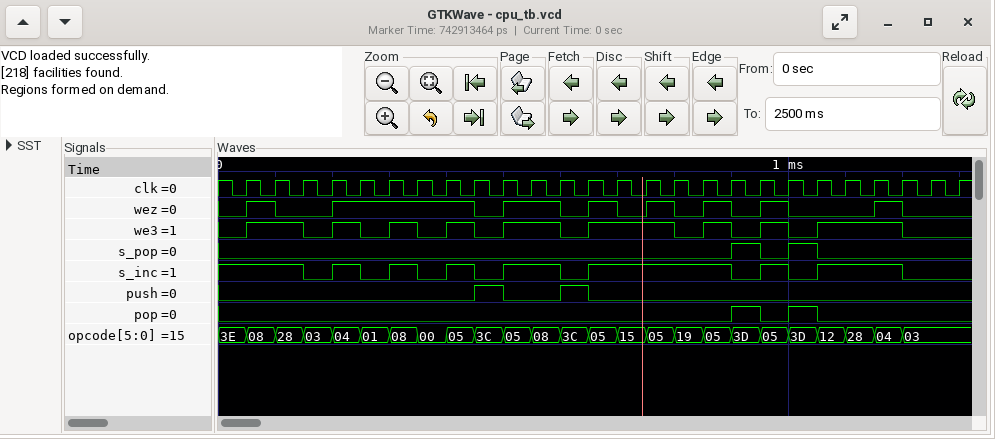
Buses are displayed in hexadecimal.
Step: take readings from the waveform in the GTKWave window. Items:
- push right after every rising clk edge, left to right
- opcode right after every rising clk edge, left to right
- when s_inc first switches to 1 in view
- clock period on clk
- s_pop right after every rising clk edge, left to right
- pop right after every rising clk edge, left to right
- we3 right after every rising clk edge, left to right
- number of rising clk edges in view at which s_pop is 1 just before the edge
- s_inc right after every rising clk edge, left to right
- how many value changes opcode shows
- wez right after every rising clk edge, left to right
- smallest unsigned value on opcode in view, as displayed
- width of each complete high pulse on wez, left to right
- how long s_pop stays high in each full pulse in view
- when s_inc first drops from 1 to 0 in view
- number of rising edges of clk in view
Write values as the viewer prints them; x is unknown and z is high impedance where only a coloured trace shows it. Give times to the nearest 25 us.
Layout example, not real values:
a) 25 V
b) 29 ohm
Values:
a) 0 0 0 0 0 0 0 0 1 0 0 1 0 0 0 0 0 0 0 0 0 0 0 0 0 0
b) 08, 28, 03, 04, 01, 08, 00, 05, 3C, 05, 08, 3C, 05, 15, 05, 19, 05, 3D, 05, 3D, 12, 28, 04, 03, 03, 03
c) 200 us
d) 50 us
e) 0 0 0 0 0 0 0 0 0 0 0 0 0 0 0 0 0 1 0 1 0 0 0 0 0 0
f) 0 0 0 0 0 0 0 0 0 0 0 0 0 0 0 0 0 1 0 1 0 0 0 0 0 0
g) 1 1 0 1 0 1 0 1 0 1 1 0 1 1 1 0 1 0 1 0 1 1 1 0 0 0
h) 2
i) 1 1 0 1 0 1 0 1 0 1 1 0 1 1 1 1 1 0 1 0 1 1 1 0 0 0
j) 24
k) 1 0 0 1 1 1 1 1 0 1 1 0 1 0 1 0 1 0 1 0 0 0 1 0 0 0
l) 00
m) 50 us, 250 us, 100 us, 50 us, 50 us, 50 us, 50 us, 50 us
n) 50 us, 50 us
o) 150 us
p) 26
